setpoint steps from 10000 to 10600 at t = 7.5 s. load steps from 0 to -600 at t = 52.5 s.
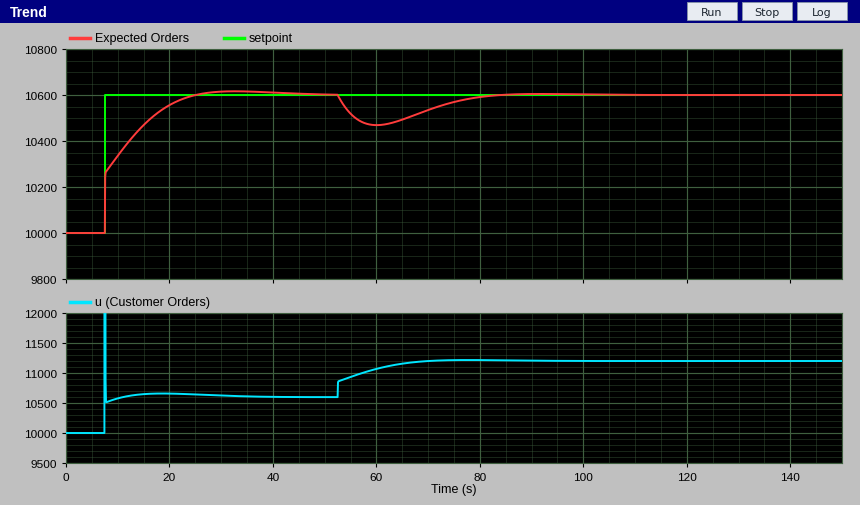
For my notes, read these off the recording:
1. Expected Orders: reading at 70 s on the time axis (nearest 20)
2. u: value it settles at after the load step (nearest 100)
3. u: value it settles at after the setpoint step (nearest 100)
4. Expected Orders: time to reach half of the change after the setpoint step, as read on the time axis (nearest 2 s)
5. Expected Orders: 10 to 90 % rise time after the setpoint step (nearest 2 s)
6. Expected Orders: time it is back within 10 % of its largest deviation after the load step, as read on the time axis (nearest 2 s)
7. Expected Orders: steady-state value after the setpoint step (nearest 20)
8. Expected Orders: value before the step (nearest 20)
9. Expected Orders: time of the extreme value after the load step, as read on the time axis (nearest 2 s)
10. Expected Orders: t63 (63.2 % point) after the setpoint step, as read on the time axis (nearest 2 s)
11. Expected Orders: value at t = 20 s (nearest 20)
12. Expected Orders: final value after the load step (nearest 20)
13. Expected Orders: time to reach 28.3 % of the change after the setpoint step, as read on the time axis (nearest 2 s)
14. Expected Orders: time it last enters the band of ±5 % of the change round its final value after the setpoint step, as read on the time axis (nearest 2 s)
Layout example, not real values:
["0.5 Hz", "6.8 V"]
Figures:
["10540", "11200", "10600", "8 s", "12 s", "78 s", "10600", "10000", "60 s", "12 s", "10560", "10600", "8 s", "22 s"]
